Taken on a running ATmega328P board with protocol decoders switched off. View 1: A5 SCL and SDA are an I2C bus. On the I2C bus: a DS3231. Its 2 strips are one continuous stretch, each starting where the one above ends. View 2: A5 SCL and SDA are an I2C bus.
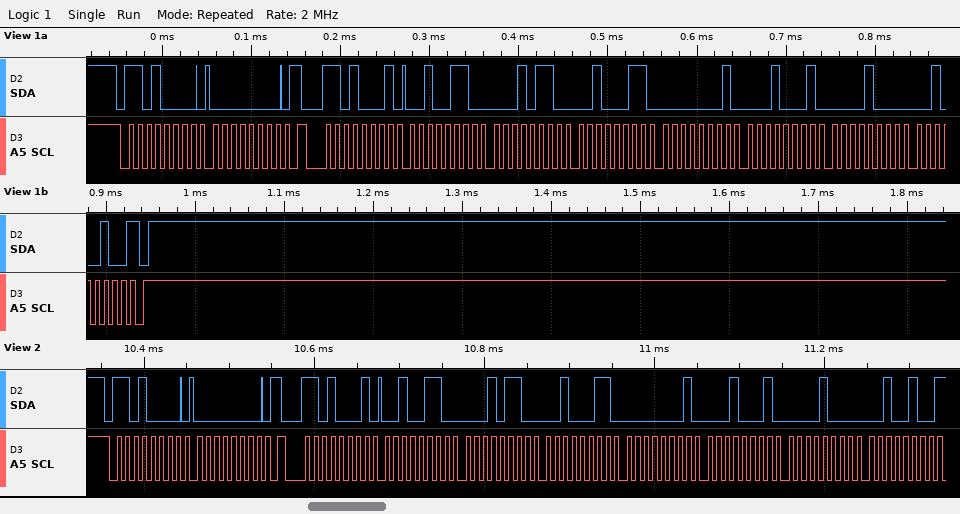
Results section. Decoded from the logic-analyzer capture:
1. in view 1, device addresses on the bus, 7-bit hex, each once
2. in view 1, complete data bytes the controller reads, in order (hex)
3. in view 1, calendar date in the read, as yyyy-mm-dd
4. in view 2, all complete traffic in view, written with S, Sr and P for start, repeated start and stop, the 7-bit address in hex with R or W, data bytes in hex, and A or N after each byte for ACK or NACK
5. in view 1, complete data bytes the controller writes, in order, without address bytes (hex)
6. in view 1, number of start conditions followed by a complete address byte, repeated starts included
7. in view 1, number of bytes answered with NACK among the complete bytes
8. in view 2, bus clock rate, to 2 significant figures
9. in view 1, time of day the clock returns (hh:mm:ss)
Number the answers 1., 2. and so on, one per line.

1. 0x68
2. 26 16 23 01 11 08 24
3. 2024-08-11
4. S 68W A 00 A Sr 68R A 26 A 16 A 23 A 01 A 11 A 08 A 24 N
5. 00
6. 2
7. 1
8. 100 kHz
9. 23:16:26
